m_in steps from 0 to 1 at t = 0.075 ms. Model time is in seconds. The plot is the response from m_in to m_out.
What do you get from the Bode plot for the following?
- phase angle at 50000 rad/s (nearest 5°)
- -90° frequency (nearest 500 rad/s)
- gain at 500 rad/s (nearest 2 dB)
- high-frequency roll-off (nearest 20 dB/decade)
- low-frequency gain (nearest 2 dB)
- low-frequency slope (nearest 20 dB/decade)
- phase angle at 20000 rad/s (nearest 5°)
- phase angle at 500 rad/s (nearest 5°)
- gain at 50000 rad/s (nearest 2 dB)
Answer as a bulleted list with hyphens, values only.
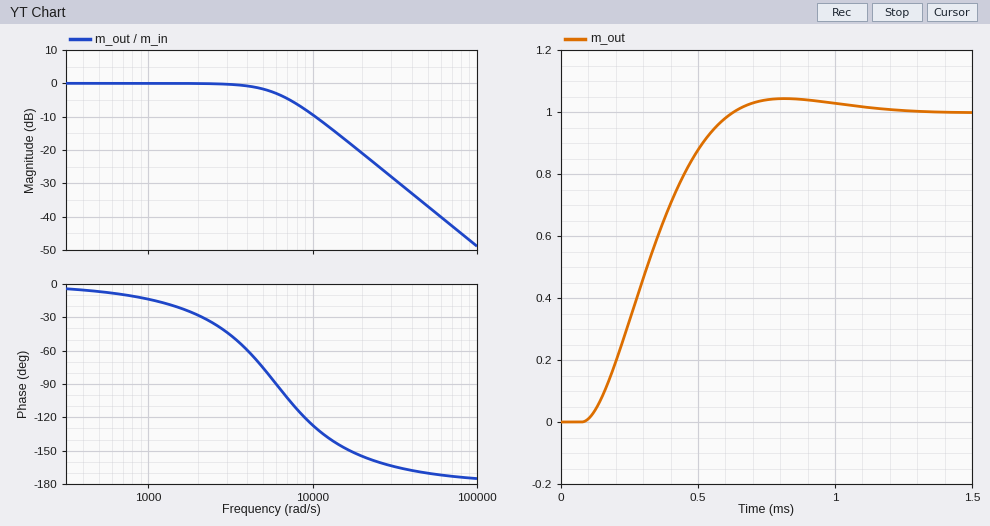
- -170°
- 6000 rad/s
- 0 dB
- -40 dB/decade
- 0 dB
- 0 dB/decade
- -155°
- -5°
- -36 dB
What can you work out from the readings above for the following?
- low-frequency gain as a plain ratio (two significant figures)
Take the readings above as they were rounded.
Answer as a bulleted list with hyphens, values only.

- 1.0
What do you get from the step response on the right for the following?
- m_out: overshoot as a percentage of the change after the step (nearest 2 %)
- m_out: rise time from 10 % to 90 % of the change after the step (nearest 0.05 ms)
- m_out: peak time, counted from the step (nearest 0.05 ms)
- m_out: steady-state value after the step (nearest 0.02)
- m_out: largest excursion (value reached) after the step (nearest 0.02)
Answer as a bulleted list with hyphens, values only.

- 4 %
- 0.35 ms
- 0.75 ms
- 1.00
- 1.04
